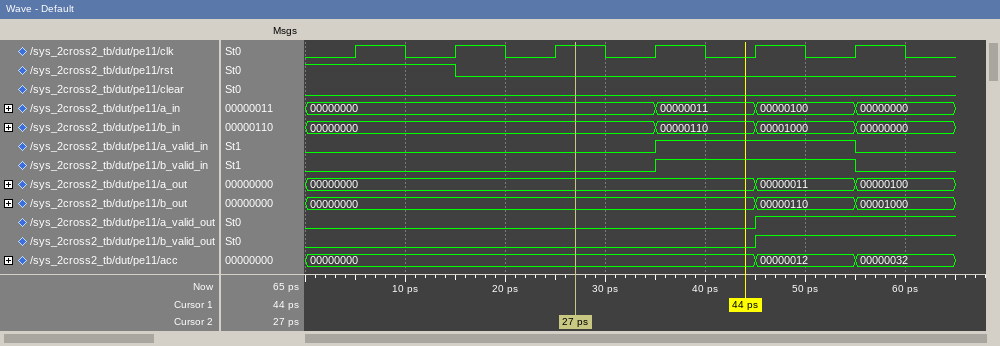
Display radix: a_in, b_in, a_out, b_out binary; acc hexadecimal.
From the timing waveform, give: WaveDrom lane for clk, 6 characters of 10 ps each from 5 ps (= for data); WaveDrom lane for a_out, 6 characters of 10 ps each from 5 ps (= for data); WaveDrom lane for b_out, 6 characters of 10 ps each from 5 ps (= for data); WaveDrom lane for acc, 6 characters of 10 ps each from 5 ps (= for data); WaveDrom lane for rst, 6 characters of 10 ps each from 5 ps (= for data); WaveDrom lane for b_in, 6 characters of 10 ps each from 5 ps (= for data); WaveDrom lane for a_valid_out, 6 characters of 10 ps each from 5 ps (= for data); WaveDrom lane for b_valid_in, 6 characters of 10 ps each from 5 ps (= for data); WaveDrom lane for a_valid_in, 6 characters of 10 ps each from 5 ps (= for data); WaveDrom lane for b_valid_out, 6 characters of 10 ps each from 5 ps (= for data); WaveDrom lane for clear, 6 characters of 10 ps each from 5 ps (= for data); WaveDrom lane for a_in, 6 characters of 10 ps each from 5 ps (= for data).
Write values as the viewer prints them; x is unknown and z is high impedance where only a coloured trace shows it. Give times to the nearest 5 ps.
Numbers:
{name: 'clk', wave: 'p.....'}
{name: 'a_out', wave: '=...==', data: '00000000 00000011 00000100'}
{name: 'b_out', wave: '=...==', data: '00000000 00000110 00001000'}
{name: 'acc', wave: '=...==', data: '00000000 00000012 00000032'}
{name: 'rst', wave: '10....'}
{name: 'b_in', wave: '=..===', data: '00000000 00000110 00001000 00000000'}
{name: 'a_valid_out', wave: '0...1.'}
{name: 'b_valid_in', wave: '0..1.0'}
{name: 'a_valid_in', wave: '0..1.0'}
{name: 'b_valid_out', wave: '0...1.'}
{name: 'clear', wave: '0.....'}
{name: 'a_in', wave: '=..===', data: '00000000 00000011 00000100 00000000'}
